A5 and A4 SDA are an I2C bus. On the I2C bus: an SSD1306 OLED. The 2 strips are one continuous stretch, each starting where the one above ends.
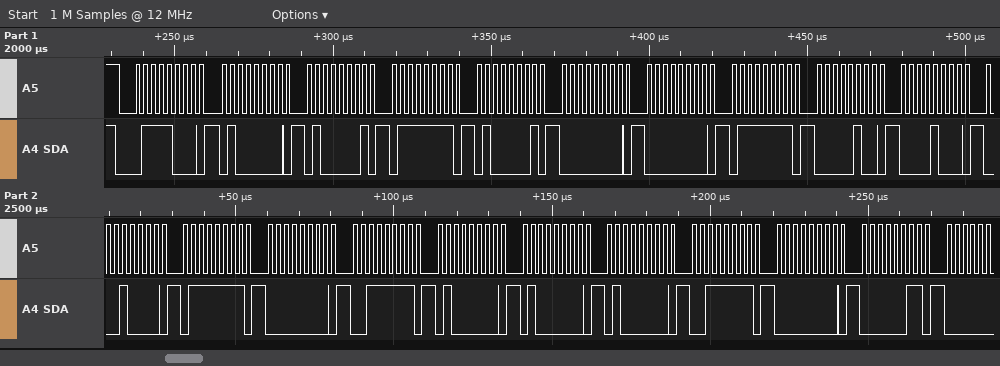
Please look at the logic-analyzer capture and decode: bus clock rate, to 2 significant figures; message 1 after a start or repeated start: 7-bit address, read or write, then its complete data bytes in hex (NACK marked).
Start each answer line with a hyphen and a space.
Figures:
- 400 kHz
- 0x3C write: 40 41 7F 41 00 00 7F 04 08 10 7F 00 3F 40 40 40 3F 00 03
